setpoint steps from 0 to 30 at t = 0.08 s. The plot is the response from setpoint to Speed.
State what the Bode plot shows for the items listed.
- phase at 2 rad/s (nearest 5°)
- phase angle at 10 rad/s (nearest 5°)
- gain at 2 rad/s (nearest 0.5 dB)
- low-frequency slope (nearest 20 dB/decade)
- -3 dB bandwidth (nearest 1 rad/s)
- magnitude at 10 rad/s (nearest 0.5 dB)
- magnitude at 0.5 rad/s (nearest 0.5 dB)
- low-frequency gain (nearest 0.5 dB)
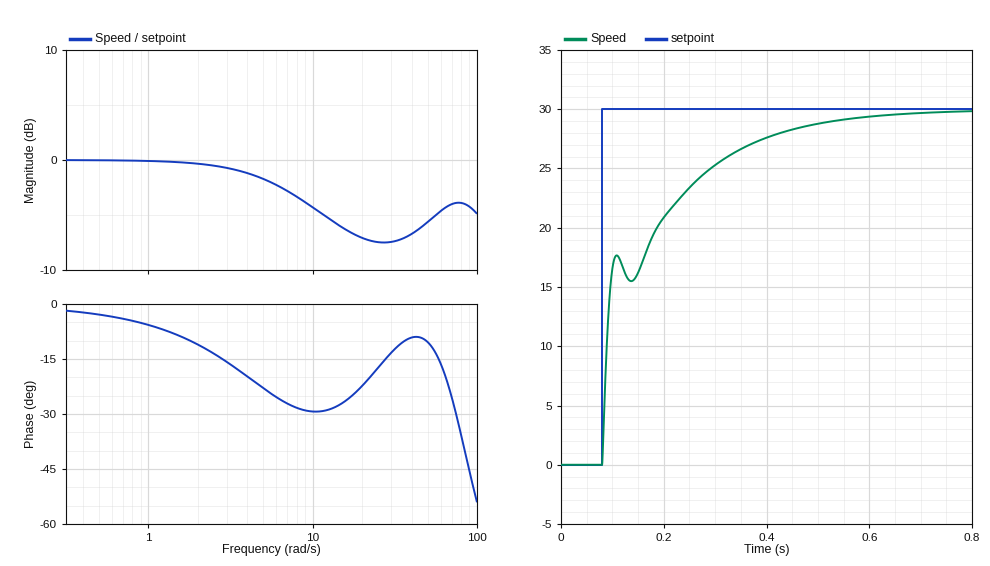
-10°
-30°
-0.5 dB
0 dB/decade
7 rad/s
-4.5 dB
0.0 dB
0.0 dB
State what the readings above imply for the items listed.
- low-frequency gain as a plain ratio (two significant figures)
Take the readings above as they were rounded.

1.0
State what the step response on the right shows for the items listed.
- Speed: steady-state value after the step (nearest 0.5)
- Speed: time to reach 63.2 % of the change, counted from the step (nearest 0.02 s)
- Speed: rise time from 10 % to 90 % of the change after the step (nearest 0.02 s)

30.0
0.10 s
0.28 s
